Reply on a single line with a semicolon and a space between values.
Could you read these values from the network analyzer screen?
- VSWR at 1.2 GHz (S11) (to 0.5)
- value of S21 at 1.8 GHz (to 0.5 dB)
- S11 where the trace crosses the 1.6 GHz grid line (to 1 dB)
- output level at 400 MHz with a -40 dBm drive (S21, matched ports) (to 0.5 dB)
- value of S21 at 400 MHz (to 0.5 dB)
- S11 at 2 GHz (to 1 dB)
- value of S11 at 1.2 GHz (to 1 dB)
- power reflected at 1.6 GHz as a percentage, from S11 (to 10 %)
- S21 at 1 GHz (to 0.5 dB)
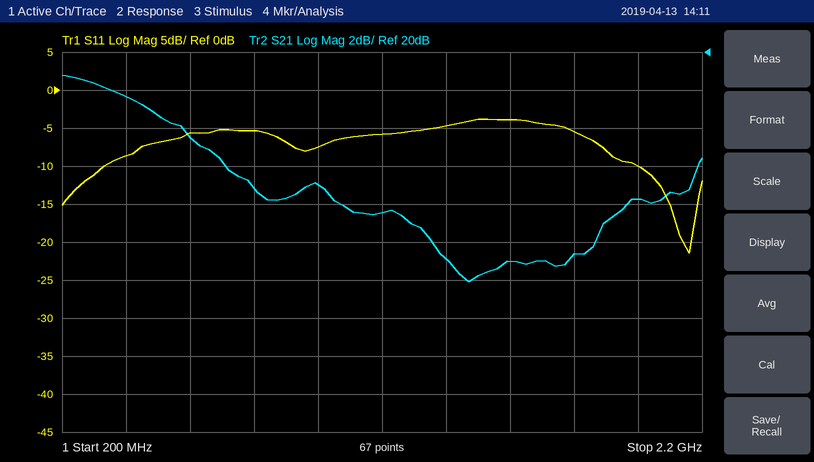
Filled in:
3.0; 9.5 dB; -4 dB; -22.5 dBm; 17.5 dB; -10 dB; -6 dB; 40 %; 13.0 dB
